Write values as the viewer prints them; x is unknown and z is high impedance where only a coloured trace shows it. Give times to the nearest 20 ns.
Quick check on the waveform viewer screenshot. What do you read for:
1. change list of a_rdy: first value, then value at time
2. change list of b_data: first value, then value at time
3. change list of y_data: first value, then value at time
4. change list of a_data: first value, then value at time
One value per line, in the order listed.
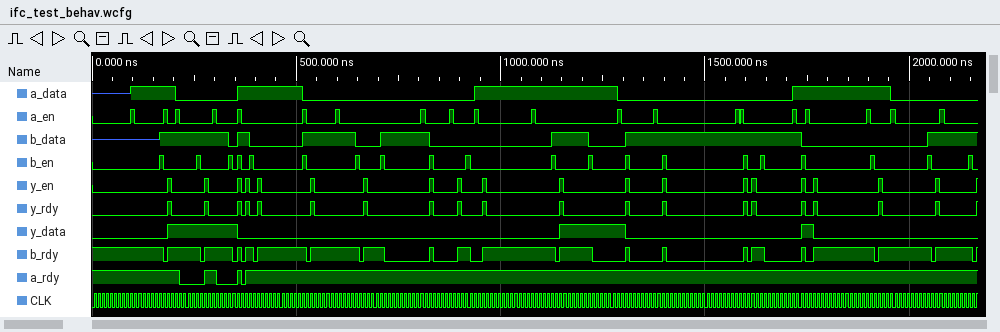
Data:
1, 0 at 220 ns, 1 at 280 ns, 0 at 300 ns, 1 at 360 ns, 0 at 360 ns, 1 at 380 ns
z, 1 at 160 ns, 0 at 340 ns, 1 at 360 ns, 0 at 380 ns, 1 at 520 ns, 0 at 640 ns, 1 at 700 ns, 0 at 820 ns, 1 at 1120 ns, 0 at 1220 ns, 1 at 1300 ns, 0 at 1740 ns, 1 at 2040 ns
0, 1 at 180 ns, 0 at 360 ns, 1 at 1140 ns, 0 at 1300 ns, 1 at 1740 ns, 0 at 1760 ns
z, 1 at 100 ns, 0 at 200 ns, 1 at 360 ns, 0 at 520 ns, 1 at 940 ns, 0 at 1280 ns, 1 at 1720 ns, 0 at 1960 ns
